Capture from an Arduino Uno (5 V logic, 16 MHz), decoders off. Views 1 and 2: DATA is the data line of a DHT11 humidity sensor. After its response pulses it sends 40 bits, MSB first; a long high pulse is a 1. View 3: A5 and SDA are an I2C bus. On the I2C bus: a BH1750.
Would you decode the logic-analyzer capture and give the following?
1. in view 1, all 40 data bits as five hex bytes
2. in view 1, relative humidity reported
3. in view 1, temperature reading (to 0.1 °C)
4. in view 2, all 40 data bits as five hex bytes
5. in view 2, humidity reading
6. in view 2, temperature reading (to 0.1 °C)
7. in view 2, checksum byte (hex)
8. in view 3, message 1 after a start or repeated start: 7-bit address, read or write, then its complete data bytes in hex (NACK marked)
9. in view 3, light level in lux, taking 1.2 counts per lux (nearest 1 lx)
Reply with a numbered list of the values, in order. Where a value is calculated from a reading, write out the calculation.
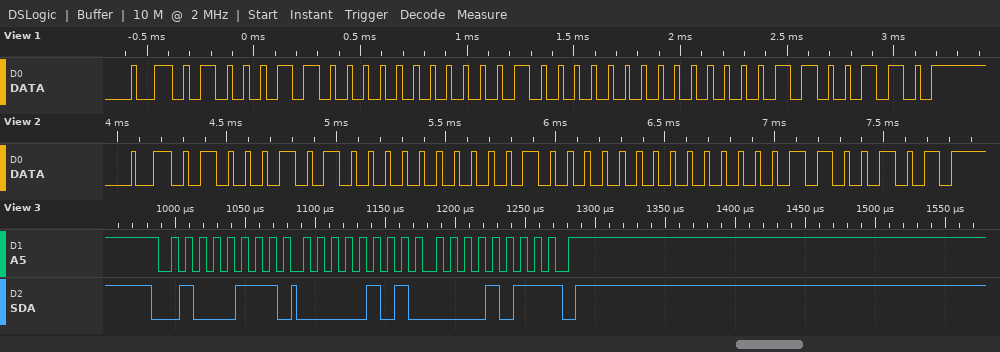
1. 46 00 20 00 66
2. 70 %
3. 32.0 °C
4. 45 00 20 00 65
5. 69 %
6. 32.0 °C
7. 0x65
8. 0x23 read: 05 0B NACK
9. 1291 / 1.2 = 1076 lx
